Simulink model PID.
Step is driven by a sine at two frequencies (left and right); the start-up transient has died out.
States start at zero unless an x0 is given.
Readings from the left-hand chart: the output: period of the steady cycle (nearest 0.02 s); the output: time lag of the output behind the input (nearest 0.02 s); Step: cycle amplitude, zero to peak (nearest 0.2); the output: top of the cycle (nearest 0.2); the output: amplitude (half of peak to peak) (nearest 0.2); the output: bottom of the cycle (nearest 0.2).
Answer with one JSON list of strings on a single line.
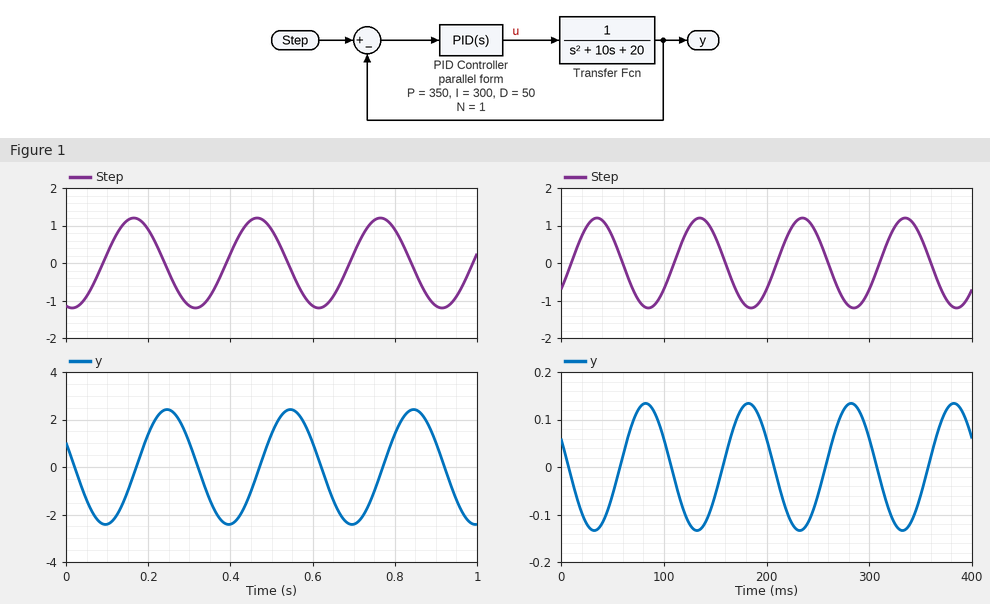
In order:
["0.30 s", "0.08 s", "1.2", "2.4", "2.4", "-2.4"]
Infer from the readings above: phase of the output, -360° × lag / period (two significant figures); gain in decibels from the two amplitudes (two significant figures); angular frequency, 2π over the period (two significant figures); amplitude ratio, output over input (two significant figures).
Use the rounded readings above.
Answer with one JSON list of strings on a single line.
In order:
["-96°", "6.0 dB", "21 rad/s", "2.0"]
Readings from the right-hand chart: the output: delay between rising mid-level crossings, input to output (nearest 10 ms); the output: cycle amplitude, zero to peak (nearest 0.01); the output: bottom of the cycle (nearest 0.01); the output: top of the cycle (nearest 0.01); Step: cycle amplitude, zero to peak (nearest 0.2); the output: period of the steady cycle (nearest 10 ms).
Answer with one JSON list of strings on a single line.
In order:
["50 ms", "0.13", "-0.13", "0.13", "1.2", "100 ms"]
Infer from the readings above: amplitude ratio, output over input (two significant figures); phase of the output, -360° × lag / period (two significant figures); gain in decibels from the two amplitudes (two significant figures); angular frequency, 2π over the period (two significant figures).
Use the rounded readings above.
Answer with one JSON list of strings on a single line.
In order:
["0.11", "-180°", "-19 dB", "0.063 rad/ms"]
